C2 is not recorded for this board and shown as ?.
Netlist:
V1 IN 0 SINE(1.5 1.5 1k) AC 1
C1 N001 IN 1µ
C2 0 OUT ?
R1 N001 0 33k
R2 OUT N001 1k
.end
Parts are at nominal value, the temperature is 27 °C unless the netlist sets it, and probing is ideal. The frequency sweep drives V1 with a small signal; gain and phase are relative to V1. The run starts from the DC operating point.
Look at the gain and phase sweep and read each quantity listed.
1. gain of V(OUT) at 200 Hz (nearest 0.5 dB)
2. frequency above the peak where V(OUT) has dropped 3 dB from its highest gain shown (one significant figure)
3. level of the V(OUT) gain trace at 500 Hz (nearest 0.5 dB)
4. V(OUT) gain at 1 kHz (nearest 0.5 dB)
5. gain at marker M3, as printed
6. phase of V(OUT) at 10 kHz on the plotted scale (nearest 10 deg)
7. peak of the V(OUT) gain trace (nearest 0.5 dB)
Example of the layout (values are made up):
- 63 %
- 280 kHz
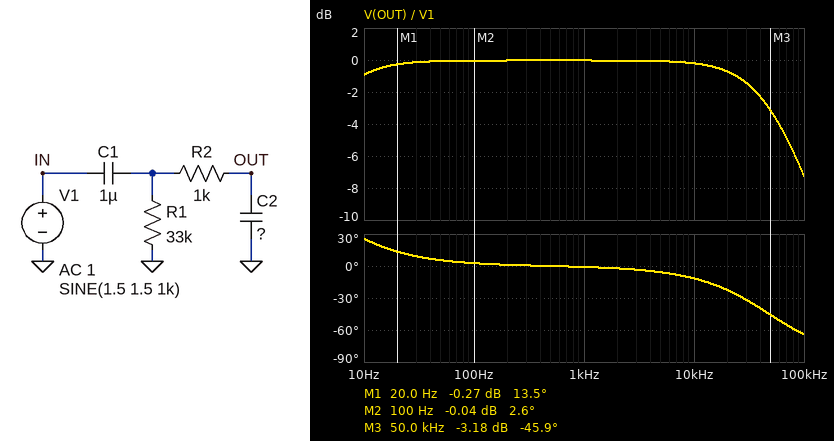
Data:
- 0 dB
- 50 kHz
- 0 dB
- 0 dB
- -3.18 dB
- -10 deg
- 0 dB
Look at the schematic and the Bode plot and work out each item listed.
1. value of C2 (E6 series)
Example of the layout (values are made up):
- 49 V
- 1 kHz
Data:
- 3.3 nF
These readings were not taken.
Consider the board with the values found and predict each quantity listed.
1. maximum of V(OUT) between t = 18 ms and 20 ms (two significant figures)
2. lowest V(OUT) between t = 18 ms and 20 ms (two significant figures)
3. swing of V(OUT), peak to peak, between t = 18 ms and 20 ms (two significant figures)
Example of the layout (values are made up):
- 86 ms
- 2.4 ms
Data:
- 1.5 V
- -1.5 V
- 3.0 V
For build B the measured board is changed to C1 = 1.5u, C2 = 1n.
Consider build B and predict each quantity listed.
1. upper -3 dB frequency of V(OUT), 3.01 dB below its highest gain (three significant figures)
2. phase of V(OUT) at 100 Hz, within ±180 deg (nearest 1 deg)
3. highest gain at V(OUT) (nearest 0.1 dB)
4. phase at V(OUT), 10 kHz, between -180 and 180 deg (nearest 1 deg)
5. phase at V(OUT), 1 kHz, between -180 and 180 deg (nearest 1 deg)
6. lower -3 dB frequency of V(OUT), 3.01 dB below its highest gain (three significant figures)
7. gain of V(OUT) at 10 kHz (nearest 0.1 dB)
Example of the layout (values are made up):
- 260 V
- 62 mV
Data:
- 159 kHz
- 2 deg
- 0 dB
- -4 deg
- 0 deg
- 3.21 Hz
- 0 dB
